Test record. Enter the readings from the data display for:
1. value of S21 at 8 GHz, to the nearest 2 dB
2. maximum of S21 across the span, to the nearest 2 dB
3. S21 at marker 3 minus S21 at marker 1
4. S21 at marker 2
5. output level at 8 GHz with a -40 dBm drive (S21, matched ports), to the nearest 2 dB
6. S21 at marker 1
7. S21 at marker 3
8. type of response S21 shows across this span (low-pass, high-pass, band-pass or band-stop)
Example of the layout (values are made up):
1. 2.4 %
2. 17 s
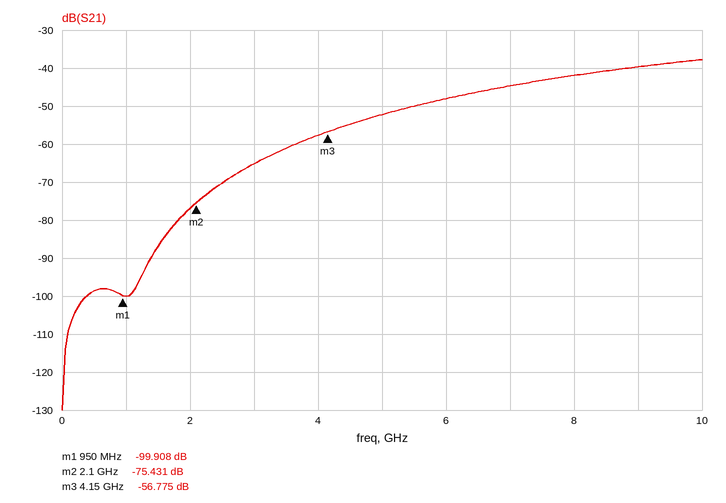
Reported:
1. -42 dB
2. -38 dB
3. 43.133 dB
4. -75.431 dB
5. -82 dBm
6. -99.908 dB
7. -56.775 dB
8. high-pass
